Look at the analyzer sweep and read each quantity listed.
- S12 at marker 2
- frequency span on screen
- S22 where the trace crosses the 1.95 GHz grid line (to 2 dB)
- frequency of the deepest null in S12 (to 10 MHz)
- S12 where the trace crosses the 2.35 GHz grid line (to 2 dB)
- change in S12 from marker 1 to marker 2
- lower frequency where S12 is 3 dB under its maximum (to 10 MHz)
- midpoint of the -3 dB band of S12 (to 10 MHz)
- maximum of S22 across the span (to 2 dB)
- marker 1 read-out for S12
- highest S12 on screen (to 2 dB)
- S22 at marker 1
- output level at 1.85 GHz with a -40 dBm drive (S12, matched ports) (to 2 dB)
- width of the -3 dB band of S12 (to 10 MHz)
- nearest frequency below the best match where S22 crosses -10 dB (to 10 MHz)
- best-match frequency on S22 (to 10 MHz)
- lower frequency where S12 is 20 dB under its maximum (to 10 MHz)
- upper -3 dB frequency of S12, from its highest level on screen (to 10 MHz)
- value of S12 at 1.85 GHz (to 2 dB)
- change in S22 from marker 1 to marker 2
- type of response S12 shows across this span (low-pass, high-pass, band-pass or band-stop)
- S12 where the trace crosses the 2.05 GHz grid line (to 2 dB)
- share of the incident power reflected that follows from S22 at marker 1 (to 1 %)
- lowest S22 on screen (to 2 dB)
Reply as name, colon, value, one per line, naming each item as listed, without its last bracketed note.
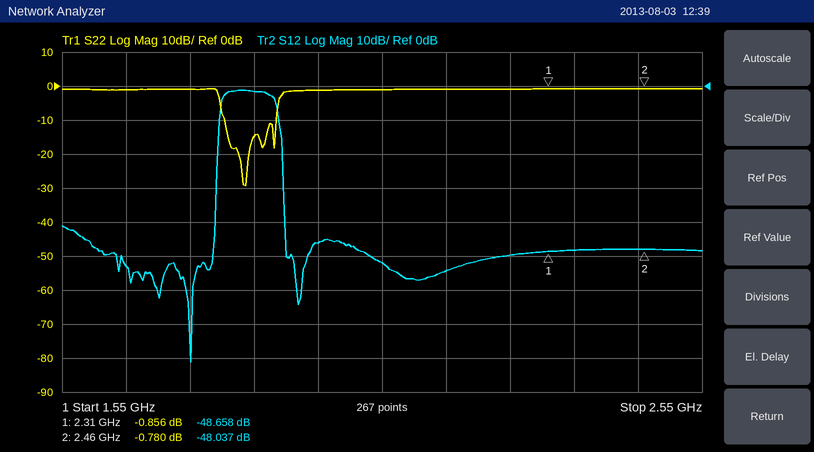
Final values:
S12 at marker 2: -48.037 dB
frequency span on screen: 1 GHz
S22 where the trace crosses the 1.95 GHz grid line: -2 dB
frequency of the deepest null in S12: 1.75 GHz
S12 where the trace crosses the 2.35 GHz grid line: -48 dB
change in S12 from marker 1 to marker 2: 0.621 dB
lower frequency where S12 is 3 dB under its maximum: 1.80 GHz
midpoint of the -3 dB band of S12: 1.84 GHz
maximum of S22 across the span: 0 dB
marker 1 read-out for S12: -48.658 dB
highest S12 on screen: -2 dB
S22 at marker 1: -0.856 dB
output level at 1.85 GHz with a -40 dBm drive (S12, matched ports): -42 dBm
width of the -3 dB band of S12: 80 MHz
nearest frequency below the best match where S22 crosses -10 dB: 1.80 GHz
best-match frequency on S22: 1.84 GHz
lower frequency where S12 is 20 dB under its maximum: 1.79 GHz
upper -3 dB frequency of S12, from its highest level on screen: 1.88 GHz
value of S12 at 1.85 GHz: -2 dB
change in S22 from marker 1 to marker 2: 0.076 dB
type of response S12 shows across this span: band-pass
S12 where the trace crosses the 2.05 GHz grid line: -52 dB
share of the incident power reflected that follows from S22 at marker 1: 82 %
lowest S22 on screen: -30 dB
